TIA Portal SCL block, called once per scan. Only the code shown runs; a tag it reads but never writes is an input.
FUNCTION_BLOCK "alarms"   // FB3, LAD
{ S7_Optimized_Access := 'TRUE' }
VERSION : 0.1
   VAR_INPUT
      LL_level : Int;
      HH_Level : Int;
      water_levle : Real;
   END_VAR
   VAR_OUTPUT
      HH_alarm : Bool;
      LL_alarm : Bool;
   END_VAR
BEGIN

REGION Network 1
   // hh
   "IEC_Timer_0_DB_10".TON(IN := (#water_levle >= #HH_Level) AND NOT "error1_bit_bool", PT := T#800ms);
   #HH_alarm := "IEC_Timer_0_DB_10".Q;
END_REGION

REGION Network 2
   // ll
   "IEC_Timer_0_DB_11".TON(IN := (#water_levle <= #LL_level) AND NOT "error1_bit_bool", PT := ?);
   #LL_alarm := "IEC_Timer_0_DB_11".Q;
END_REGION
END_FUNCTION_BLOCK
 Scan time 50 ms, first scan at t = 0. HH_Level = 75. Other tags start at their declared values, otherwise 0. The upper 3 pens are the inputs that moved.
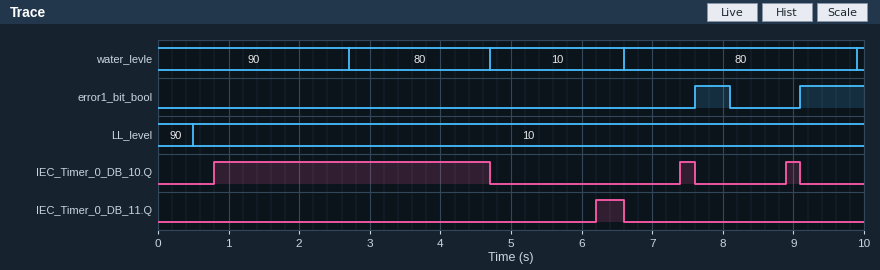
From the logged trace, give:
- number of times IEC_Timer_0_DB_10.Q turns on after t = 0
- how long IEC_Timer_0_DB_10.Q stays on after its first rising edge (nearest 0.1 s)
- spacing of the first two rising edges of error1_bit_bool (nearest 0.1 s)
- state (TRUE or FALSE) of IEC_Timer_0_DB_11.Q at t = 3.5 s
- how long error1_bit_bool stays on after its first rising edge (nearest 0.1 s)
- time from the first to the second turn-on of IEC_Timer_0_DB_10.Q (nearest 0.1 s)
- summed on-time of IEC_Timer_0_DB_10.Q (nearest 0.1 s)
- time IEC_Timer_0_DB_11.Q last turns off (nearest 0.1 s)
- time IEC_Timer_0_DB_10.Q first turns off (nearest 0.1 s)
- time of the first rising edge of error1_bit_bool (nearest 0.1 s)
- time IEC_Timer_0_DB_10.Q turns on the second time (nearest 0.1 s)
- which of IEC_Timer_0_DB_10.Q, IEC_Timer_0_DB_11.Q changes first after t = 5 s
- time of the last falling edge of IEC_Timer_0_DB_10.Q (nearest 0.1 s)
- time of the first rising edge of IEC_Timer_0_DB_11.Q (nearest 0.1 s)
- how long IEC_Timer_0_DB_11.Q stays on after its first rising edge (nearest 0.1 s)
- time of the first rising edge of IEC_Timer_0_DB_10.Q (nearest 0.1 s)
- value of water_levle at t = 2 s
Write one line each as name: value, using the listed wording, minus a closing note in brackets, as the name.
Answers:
number of times IEC_Timer_0_DB_10.Q turns on after t = 0: 3
how long IEC_Timer_0_DB_10.Q stays on after its first rising edge: 3.9 s
spacing of the first two rising edges of error1_bit_bool: 1.5 s
state (TRUE or FALSE) of IEC_Timer_0_DB_11.Q at t = 3.5 s: FALSE
how long error1_bit_bool stays on after its first rising edge: 0.5 s
time from the first to the second turn-on of IEC_Timer_0_DB_10.Q: 6.6 s
summed on-time of IEC_Timer_0_DB_10.Q: 4.3 s
time IEC_Timer_0_DB_11.Q last turns off: 6.6 s
time IEC_Timer_0_DB_10.Q first turns off: 4.7 s
time of the first rising edge of error1_bit_bool: 7.6 s
time IEC_Timer_0_DB_10.Q turns on the second time: 7.4 s
which of IEC_Timer_0_DB_10.Q, IEC_Timer_0_DB_11.Q changes first after t = 5 s: IEC_Timer_0_DB_11.Q
time of the last falling edge of IEC_Timer_0_DB_10.Q: 9.1 s
time of the first rising edge of IEC_Timer_0_DB_11.Q: 6.2 s
how long IEC_Timer_0_DB_11.Q stays on after its first rising edge: 0.4 s
time of the first rising edge of IEC_Timer_0_DB_10.Q: 0.8 s
value of water_levle at t = 2 s: 90
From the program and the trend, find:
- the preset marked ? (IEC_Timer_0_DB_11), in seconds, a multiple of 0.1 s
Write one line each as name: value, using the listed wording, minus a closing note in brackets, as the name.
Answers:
the preset marked ? (IEC_Timer_0_DB_11), in seconds, a multiple of 0.1 s: 1.5 s
